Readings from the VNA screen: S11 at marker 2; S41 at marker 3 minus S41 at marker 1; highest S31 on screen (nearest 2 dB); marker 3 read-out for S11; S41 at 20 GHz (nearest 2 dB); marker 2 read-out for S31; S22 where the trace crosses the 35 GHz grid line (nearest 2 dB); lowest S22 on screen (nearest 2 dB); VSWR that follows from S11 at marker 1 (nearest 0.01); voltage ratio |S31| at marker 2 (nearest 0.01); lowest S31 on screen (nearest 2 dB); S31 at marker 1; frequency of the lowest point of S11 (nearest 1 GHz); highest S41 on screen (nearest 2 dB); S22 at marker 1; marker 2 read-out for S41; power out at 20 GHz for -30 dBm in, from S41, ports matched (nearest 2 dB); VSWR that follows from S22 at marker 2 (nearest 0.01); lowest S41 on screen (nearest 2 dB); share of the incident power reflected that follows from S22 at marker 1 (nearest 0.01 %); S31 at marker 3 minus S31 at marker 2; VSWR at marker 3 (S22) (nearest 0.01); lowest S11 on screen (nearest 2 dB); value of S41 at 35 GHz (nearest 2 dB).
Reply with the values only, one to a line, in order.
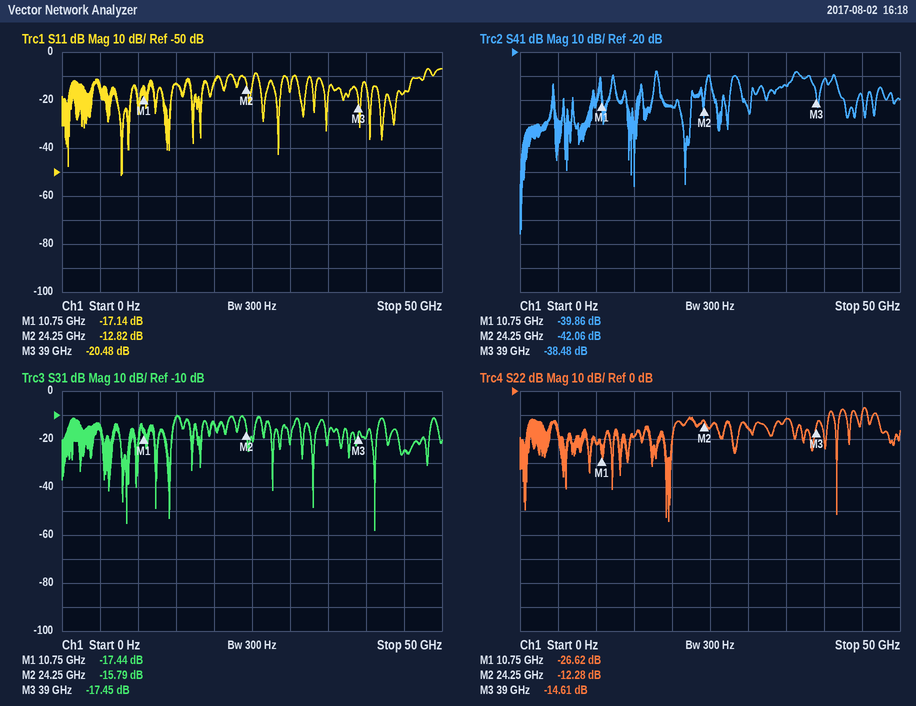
-12.82 dB
1.38 dB
-10 dB
-20.48 dB
-42 dB
-15.79 dB
-12 dB
-54 dB
1.32
0.16
-58 dB
-17.44 dB
8 GHz
-28 dB
-26.62 dB
-42.06 dB
-72 dBm
1.64
-96 dB
0.22 %
-1.66 dB
1.46
-52 dB
-34 dB
